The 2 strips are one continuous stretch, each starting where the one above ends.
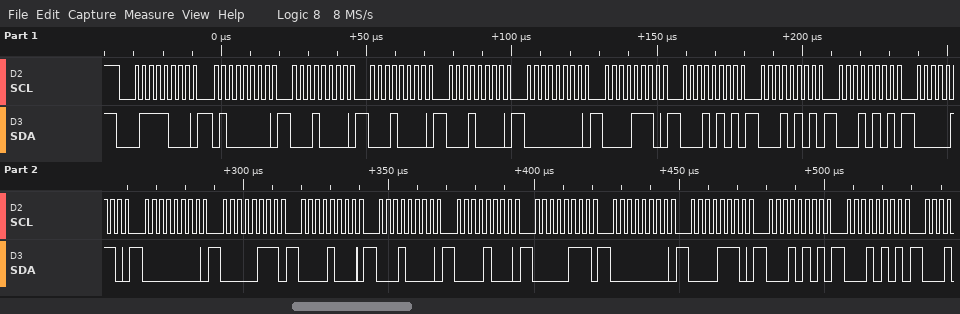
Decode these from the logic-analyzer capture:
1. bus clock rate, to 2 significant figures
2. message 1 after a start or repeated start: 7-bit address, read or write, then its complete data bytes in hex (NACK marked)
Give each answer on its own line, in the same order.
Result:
400 kHz
0x3C write: 40 10 10 10 00 0E 15 15 15 06 00 07 08 10 08 07 00 0E 15 15
